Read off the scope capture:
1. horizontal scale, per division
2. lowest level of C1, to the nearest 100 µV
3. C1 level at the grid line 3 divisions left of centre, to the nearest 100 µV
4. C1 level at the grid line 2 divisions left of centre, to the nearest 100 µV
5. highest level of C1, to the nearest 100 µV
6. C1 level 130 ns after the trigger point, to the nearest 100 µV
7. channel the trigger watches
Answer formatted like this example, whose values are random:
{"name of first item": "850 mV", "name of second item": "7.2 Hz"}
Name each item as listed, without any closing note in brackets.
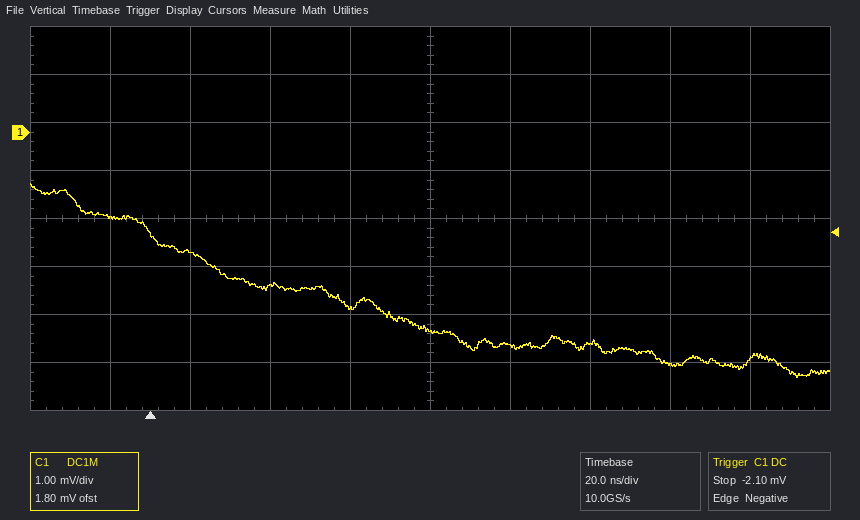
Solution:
{"horizontal scale, per division": "20 ns", "lowest level of C1, to the nearest 100 µV": "-5.1 mV", "C1 level at the grid line 3 divisions left of centre, to the nearest 100 µV": "-2.5 mV", "C1 level at the grid line 2 divisions left of centre, to the nearest 100 µV": "-3.2 mV", "highest level of C1, to the nearest 100 µV": "-1.1 mV", "C1 level 130 ns after the trigger point, to the nearest 100 µV": "-4.8 mV", "channel the trigger watches": "C1"}
